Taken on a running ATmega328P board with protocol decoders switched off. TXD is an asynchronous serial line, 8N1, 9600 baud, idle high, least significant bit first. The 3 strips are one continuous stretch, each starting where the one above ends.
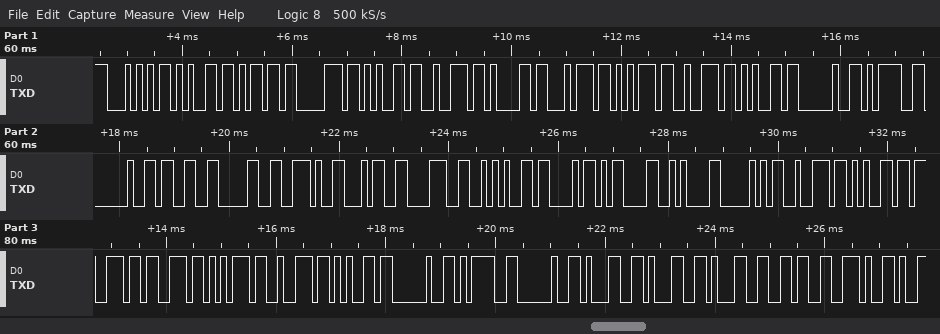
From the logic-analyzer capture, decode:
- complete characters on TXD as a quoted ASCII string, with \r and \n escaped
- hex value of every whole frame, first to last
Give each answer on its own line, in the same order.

"Temperature = 30.48*C\r\nPressure = 1116."
0x54 0x65 0x6D 0x70 0x65 0x72 0x61 0x74 0x75 0x72 0x65 0x20 0x3D 0x20 0x33 0x30 0x2E 0x34 0x38 0x2A 0x43 0x0D 0x0A 0x50 0x72 0x65 0x73 0x73 0x75 0x72 0x65 0x20 0x3D 0x20 0x31 0x31 0x31 0x36 0x2E
